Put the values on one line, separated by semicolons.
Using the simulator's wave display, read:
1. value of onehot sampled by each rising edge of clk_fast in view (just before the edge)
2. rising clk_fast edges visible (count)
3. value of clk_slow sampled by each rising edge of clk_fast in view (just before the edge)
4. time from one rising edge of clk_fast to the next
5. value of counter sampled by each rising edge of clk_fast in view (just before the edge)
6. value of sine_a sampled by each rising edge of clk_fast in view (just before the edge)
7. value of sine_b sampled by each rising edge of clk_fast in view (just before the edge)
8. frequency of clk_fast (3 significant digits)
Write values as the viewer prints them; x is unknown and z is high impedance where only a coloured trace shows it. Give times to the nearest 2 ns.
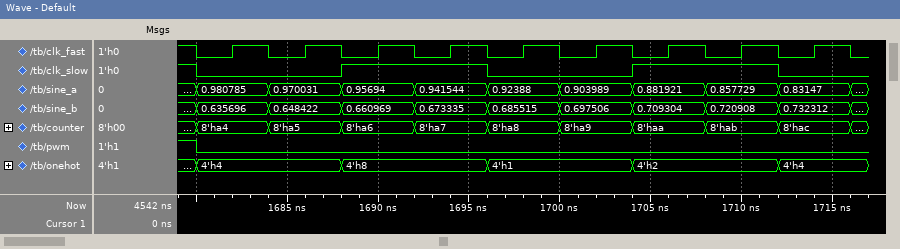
4'h4, 4'h4, 4'h8, 4'h8, 4'h1, 4'h1, 4'h2, 4'h2, 4'h4; 9; 0 0 1 1 0 0 1 1 0; 4 ns; 8'ha4, 8'ha5, 8'ha6, 8'ha7, 8'ha8, 8'ha9, 8'haa, 8'hab, 8'hac; 0.980785, 0.970031, 0.95694, 0.941544, 0.92388, 0.903989, 0.881921, 0.857729, 0.83147; 0.635696, 0.648422, 0.660969, 0.673335, 0.685515, 0.697506, 0.709304, 0.720908, 0.732312; 250 MHz
